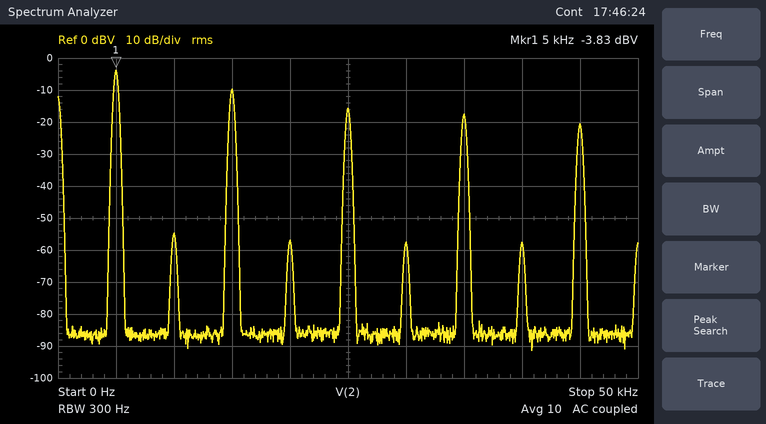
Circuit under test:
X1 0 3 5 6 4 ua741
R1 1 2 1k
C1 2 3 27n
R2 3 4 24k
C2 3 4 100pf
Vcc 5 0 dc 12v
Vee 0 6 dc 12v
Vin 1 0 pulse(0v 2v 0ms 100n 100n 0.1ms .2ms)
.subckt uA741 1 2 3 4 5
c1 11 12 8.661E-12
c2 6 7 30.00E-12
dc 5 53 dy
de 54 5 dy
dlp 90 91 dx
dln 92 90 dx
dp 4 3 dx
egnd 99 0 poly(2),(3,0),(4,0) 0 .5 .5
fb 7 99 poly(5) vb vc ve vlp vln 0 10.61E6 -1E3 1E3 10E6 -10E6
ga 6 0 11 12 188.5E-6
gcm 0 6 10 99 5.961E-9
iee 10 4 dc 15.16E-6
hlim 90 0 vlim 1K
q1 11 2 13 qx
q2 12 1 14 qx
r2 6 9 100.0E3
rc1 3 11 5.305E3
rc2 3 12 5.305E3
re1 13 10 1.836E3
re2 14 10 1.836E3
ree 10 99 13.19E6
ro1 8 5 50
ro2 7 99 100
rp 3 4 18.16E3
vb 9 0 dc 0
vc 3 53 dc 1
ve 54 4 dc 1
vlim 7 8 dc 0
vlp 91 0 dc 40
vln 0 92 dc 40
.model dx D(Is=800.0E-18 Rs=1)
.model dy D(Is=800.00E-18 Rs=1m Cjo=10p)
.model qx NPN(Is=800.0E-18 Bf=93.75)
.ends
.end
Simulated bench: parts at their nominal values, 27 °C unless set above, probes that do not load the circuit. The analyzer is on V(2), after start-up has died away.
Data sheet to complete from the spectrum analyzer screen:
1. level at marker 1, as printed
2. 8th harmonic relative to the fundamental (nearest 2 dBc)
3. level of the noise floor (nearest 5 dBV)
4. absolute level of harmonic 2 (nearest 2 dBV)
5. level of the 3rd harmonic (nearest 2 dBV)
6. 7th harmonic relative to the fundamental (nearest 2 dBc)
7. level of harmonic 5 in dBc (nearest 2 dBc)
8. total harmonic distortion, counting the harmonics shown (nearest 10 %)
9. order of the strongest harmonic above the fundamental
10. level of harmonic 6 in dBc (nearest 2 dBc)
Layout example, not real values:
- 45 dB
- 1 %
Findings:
- -3.83 dBV
- -54 dBc
- -85 dBV
- -54 dBV
- -10 dBV
- -14 dBc
- -12 dBc
- 60 %
- 3
- -54 dBc
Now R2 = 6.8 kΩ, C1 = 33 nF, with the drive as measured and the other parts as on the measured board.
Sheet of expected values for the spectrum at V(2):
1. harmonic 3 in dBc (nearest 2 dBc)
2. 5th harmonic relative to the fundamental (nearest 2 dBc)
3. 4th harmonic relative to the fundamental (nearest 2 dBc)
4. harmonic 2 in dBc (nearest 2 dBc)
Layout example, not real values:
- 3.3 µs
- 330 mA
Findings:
- -8 dBc
- -8 dBc
- -50 dBc
- -60 dBc
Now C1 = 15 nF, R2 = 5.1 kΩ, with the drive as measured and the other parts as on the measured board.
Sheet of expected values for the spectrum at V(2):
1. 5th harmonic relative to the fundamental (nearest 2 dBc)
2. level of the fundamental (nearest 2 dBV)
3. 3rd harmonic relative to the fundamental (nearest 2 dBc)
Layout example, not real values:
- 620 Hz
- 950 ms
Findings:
- -18 dBc
- -2 dBV
- -20 dBc
